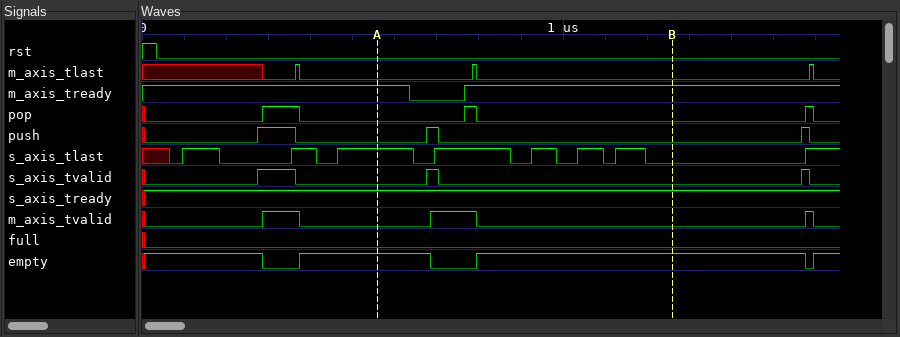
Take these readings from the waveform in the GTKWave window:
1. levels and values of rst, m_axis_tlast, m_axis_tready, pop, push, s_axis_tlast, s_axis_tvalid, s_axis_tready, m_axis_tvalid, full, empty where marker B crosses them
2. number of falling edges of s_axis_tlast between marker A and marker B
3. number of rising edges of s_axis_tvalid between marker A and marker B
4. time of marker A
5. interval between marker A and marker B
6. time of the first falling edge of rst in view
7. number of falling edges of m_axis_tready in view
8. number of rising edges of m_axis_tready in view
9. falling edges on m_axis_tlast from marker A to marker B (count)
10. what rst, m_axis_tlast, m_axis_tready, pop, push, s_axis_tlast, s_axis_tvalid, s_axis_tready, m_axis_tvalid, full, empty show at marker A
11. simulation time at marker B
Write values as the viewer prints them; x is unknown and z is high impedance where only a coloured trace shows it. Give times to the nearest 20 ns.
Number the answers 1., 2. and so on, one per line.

1. rst=0, m_axis_tlast=0, m_axis_tready=1, pop=0, push=0, s_axis_tlast=0, s_axis_tvalid=0, s_axis_tready=1, m_axis_tvalid=0, full=0, empty=1
2. 5
3. 1
4. 560 ns
5. 700 ns
6. 40 ns
7. 1
8. 1
9. 1
10. rst=0, m_axis_tlast=0, m_axis_tready=1, pop=0, push=0, s_axis_tlast=1, s_axis_tvalid=0, s_axis_tready=1, m_axis_tvalid=0, full=0, empty=1
11. 1260 ns
